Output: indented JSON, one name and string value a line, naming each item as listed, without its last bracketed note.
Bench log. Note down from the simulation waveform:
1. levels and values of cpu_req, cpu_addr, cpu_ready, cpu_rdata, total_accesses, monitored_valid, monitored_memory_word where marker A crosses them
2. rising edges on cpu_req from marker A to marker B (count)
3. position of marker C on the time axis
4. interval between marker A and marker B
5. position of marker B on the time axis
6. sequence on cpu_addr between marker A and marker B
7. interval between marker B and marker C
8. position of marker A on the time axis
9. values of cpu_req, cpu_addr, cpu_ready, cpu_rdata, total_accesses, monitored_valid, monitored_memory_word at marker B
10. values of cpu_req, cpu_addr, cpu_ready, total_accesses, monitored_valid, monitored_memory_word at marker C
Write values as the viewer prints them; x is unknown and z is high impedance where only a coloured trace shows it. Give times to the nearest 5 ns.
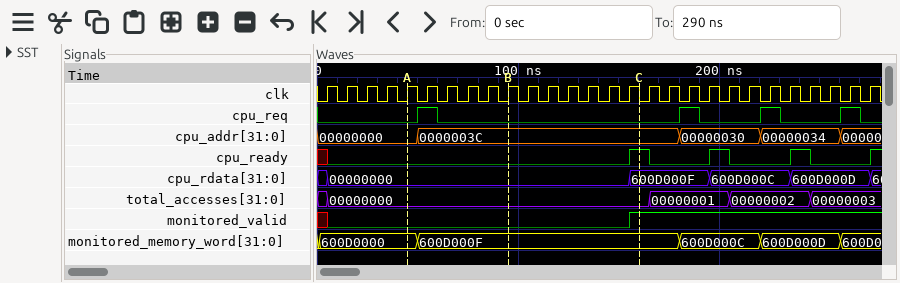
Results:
{
  "levels and values of cpu_req, cpu_addr, cpu_ready, cpu_rdata, total_accesses, monitored_valid, monitored_memory_word where marker A crosses them": "cpu_req=0, cpu_addr=00000000, cpu_ready=0, cpu_rdata=00000000, total_accesses=00000000, monitored_valid=0, monitored_memory_word=600D0000",
  "rising edges on cpu_req from marker A to marker B": "1",
  "position of marker C on the time axis": "160 ns",
  "interval between marker A and marker B": "50 ns",
  "position of marker B on the time axis": "95 ns",
  "sequence on cpu_addr between marker A and marker B": "00000000, 0000003C",
  "interval between marker B and marker C": "65 ns",
  "position of marker A on the time axis": "45 ns",
  "values of cpu_req, cpu_addr, cpu_ready, cpu_rdata, total_accesses, monitored_valid, monitored_memory_word at marker B": "cpu_req=0, cpu_addr=0000003C, cpu_ready=0, cpu_rdata=00000000, total_accesses=00000000, monitored_valid=0, monitored_memory_word=600D000F",
  "values of cpu_req, cpu_addr, cpu_ready, total_accesses, monitored_valid, monitored_memory_word at marker C": "cpu_req=0, cpu_addr=0000003C, cpu_ready=1, total_accesses=00000000, monitored_valid=1, monitored_memory_word=600D000F"
}
